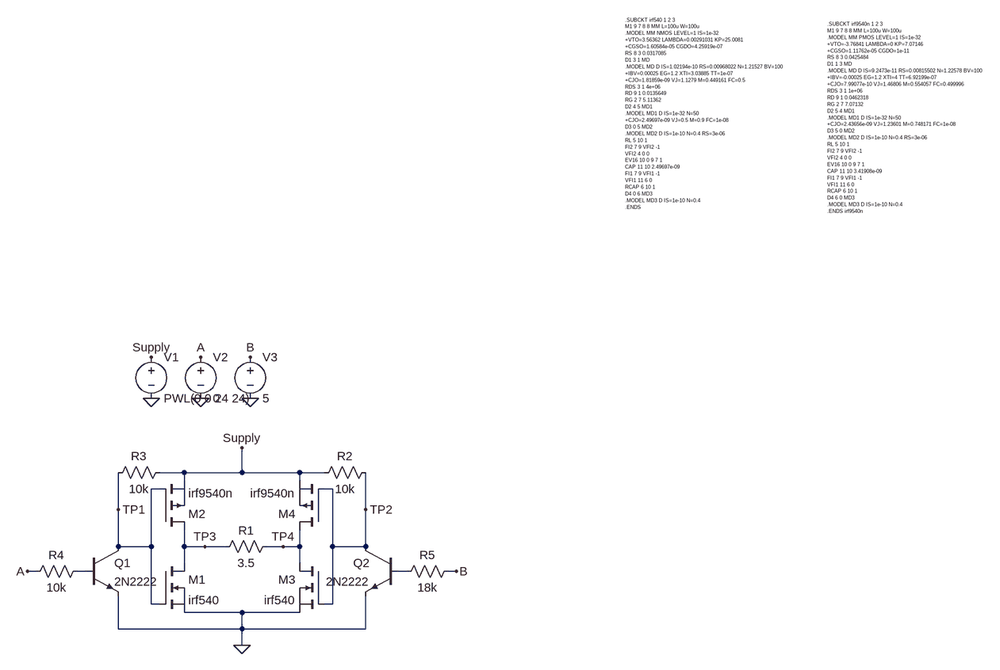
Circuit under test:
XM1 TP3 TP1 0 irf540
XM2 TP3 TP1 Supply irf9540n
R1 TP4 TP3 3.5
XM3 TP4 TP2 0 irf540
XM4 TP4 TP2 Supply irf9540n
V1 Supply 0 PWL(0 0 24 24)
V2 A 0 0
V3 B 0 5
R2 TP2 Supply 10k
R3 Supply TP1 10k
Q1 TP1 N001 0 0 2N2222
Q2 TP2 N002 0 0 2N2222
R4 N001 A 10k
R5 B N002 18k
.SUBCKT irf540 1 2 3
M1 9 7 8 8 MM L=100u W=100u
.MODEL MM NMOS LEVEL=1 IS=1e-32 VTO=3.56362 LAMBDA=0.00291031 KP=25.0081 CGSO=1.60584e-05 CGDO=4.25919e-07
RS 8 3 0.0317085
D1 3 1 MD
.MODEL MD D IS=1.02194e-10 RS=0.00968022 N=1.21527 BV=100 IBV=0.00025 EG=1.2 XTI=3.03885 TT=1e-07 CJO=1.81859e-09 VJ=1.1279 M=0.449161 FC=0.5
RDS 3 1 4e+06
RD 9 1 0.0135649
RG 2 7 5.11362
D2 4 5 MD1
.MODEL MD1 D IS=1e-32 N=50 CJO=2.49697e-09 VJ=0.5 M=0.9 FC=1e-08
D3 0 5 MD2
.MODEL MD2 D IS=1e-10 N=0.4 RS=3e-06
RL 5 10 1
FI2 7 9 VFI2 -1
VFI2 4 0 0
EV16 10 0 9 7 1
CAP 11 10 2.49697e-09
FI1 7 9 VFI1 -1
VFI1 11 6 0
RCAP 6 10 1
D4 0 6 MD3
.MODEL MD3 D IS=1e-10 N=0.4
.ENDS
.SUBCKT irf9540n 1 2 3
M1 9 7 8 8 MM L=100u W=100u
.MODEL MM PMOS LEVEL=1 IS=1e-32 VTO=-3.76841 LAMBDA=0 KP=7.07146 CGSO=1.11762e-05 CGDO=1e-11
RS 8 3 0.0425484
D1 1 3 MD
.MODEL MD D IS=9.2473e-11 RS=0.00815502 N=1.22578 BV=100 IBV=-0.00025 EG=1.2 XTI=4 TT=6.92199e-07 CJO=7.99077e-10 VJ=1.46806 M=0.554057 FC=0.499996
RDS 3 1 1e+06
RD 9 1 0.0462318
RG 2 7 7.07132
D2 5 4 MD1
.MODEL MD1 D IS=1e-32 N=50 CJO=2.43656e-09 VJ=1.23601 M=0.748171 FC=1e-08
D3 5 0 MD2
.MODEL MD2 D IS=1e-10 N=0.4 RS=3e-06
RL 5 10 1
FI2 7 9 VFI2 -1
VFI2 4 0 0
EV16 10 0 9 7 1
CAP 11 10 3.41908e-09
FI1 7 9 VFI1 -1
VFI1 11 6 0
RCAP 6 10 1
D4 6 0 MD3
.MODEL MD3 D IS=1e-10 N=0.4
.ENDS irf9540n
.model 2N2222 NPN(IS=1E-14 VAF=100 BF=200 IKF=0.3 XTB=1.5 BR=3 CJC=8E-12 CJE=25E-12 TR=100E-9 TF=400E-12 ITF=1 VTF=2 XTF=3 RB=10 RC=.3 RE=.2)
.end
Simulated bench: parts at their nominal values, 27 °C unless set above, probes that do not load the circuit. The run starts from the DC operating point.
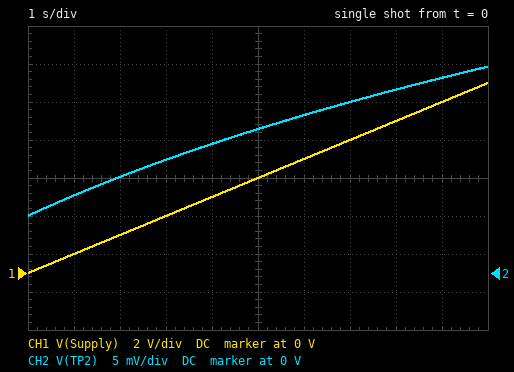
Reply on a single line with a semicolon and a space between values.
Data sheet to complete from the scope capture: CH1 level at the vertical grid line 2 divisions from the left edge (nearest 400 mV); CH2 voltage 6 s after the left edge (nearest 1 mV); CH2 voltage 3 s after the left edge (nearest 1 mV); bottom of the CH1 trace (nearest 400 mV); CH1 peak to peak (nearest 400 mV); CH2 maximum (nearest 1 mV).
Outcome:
2.0 V; 21 mV; 15 mV; 0 V; 10.0 V; 27 mV
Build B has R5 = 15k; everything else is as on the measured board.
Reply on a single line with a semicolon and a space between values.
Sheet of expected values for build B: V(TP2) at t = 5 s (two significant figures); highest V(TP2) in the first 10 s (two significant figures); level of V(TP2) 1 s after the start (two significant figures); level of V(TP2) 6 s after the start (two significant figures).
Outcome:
17 mV; 25 mV; 9.8 mV; 19 mV
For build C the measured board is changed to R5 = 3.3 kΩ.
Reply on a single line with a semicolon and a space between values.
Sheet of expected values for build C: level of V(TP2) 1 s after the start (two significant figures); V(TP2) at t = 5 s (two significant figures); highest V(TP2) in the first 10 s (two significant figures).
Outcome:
8.4 mV; 11 mV; 13 mV
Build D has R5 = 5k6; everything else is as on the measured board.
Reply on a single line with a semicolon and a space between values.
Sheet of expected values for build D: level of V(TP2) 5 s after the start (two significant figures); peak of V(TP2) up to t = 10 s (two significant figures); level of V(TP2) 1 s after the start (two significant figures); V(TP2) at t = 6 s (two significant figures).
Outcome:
12 mV; 16 mV; 8.6 mV; 13 mV
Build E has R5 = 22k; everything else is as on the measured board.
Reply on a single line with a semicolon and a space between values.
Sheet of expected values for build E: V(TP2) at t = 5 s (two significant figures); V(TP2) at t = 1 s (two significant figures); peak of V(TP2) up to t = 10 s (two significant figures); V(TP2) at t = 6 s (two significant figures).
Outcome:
21 mV; 11 mV; 30 mV; 23 mV
